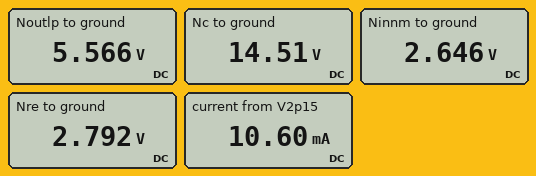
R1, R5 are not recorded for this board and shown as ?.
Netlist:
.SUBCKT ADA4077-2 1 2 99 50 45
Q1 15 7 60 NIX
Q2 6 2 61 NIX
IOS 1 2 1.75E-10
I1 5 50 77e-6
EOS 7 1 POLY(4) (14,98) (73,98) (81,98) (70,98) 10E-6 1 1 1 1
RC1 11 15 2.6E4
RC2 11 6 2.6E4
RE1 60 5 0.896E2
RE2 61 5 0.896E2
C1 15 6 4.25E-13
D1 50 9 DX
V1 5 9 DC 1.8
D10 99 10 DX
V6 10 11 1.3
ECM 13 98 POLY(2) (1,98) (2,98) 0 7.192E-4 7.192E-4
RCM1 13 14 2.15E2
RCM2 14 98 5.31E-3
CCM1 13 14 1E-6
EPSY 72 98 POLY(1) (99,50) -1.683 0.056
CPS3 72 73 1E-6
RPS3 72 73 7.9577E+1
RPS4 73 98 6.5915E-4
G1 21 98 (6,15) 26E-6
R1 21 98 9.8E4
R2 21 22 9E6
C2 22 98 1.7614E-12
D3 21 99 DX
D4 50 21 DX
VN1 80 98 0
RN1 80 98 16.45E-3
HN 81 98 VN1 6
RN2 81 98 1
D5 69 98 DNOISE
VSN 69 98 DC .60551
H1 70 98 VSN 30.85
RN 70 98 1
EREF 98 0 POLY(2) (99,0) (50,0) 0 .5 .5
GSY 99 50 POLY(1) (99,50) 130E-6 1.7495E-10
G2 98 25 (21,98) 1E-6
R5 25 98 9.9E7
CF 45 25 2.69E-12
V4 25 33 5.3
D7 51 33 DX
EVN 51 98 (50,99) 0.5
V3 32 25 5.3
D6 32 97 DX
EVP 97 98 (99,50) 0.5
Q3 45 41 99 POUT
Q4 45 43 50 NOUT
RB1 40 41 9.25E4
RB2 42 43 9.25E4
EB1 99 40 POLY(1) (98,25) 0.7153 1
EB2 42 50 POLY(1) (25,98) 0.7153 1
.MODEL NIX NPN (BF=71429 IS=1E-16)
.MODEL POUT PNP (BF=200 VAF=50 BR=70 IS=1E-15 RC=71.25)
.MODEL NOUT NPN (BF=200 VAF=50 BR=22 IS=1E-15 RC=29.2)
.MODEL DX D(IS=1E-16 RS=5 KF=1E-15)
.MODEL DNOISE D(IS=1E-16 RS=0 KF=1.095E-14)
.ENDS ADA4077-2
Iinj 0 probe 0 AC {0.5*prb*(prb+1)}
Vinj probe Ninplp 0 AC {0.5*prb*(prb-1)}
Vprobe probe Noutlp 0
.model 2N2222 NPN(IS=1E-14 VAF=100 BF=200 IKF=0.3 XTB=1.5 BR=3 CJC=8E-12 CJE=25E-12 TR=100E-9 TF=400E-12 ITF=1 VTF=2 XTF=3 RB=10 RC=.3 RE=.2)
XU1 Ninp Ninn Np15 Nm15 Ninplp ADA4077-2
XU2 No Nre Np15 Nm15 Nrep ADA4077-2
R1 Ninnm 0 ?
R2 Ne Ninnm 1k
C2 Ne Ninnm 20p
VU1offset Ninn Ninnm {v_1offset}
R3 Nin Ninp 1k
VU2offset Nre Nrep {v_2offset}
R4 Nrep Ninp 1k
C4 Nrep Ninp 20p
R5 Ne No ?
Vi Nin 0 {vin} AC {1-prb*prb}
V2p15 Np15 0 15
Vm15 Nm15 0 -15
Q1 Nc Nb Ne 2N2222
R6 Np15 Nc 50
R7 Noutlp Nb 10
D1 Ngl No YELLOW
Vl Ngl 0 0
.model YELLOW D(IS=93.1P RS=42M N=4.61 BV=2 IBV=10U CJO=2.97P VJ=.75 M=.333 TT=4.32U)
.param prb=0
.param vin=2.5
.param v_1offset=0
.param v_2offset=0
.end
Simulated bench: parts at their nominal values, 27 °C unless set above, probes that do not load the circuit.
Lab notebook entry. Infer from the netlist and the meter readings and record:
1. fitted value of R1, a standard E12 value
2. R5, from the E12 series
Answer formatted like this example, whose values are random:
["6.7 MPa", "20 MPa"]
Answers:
["1.2 kΩ", "270 Ω"]
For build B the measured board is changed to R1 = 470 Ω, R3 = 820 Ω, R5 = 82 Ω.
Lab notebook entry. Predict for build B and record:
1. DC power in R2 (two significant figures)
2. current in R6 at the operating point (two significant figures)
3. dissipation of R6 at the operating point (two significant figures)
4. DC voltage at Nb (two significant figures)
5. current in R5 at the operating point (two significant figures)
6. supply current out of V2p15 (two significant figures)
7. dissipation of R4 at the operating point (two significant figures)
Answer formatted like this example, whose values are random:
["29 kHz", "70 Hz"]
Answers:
["34 mW", "73 mA", "270 mW", "9.4 V", "68 mA", "74 mA", "93 µW"]
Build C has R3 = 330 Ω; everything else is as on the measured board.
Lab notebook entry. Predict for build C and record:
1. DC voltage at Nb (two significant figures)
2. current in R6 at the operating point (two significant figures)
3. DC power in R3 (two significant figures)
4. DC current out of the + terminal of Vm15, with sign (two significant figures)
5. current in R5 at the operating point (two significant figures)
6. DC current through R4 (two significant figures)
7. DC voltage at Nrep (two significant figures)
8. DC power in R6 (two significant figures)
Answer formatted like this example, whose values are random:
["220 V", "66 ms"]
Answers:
["5.4 V", "9.2 mA", "15 µW", "-600 µA", "7.1 mA", "210 µA", "2.8 V", "4.3 mW"]
